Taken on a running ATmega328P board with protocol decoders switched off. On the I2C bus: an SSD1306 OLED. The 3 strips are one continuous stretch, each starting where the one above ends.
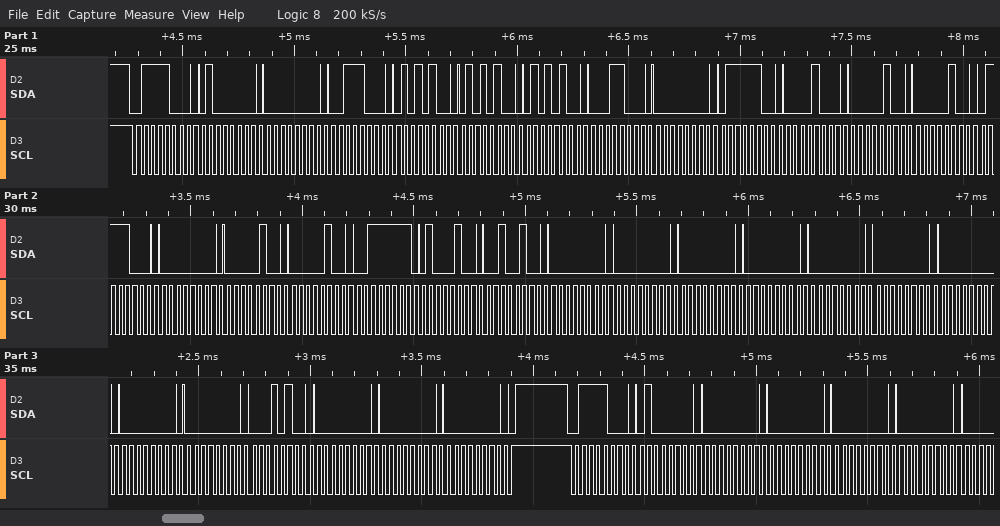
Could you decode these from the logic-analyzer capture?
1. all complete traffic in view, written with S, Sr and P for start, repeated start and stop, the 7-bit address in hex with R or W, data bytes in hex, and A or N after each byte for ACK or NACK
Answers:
S 3CW A 40 A 00 A 38 A 54 A 54 A 54 A 18 A 00 A 7C A 08 A 04 A 04 A 78 A 00 A 04 A 04 A 3F A 44 A 24 A 00 A 00 A 00 A 00 A 00 A 00 A 00 A 00 A 00 A 14 A 00 A 00 A 00 A P S 3CW A 40 A 00 A 00 A 00 A 00 A
